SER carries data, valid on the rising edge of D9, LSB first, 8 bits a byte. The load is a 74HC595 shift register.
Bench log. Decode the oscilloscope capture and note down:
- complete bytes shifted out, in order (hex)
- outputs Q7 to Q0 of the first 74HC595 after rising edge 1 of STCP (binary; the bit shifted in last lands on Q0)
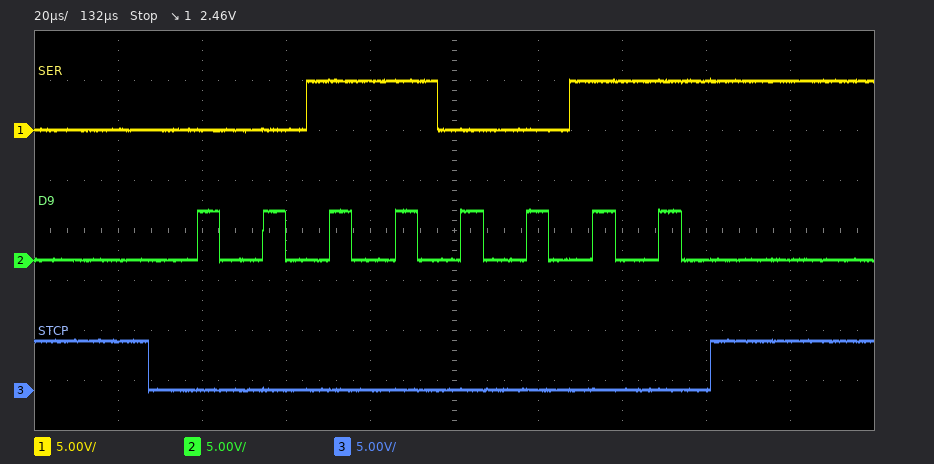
CC
00110011
